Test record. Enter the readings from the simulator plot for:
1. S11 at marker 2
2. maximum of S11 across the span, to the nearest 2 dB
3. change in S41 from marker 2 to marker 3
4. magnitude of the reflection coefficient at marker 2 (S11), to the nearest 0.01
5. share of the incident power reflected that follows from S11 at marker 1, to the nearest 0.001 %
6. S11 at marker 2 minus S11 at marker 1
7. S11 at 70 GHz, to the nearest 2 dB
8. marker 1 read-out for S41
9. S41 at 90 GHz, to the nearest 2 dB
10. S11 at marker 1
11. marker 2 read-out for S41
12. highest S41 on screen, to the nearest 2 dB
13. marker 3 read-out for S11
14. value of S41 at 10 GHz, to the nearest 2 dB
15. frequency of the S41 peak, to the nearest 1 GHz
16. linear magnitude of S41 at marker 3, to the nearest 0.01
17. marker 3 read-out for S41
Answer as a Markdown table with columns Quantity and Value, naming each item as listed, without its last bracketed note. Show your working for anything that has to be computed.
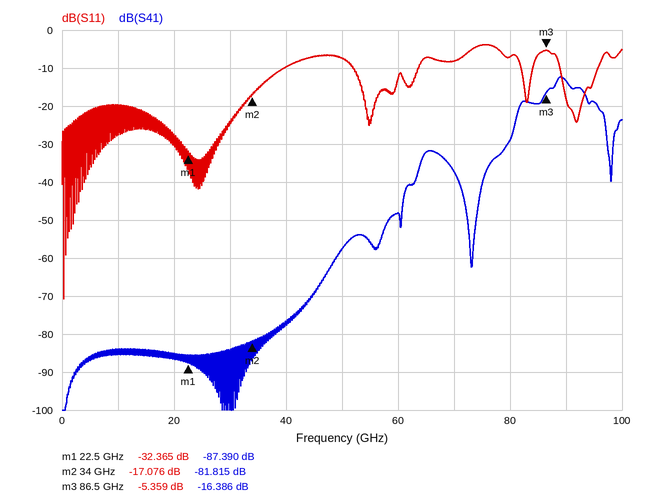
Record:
| Quantity | Value |
|---|---|
| S11 at marker 2 | -17.076 dB |
| maximum of S11 across the span, to the nearest 2 dB | -4 dB |
| change in S41 from marker 2 to marker 3 | -16.386 − (-81.815) = 65.429 dB |
| magnitude of the reflection coefficient at marker 2 (S11), to the nearest 0.01 | 10^(-17.076/20) ≈ 0.14 |
| share of the incident power reflected that follows from S11 at marker 1, to the nearest 0.001 % | 10^(-32.365/10) ≈ 0.058 % |
| S11 at marker 2 minus S11 at marker 1 | -17.076 − (-32.365) = 15.289 dB |
| S11 at 70 GHz, to the nearest 2 dB | -8 dB |
| marker 1 read-out for S41 | -87.390 dB |
| S41 at 90 GHz, to the nearest 2 dB | -14 dB |
| S11 at marker 1 | -32.365 dB |
| marker 2 read-out for S41 | -81.815 dB |
| highest S41 on screen, to the nearest 2 dB | -12 dB |
| marker 3 read-out for S11 | -5.359 dB |
| value of S41 at 10 GHz, to the nearest 2 dB | -84 dB |
| frequency of the S41 peak, to the nearest 1 GHz | 89 GHz |
| linear magnitude of S41 at marker 3, to the nearest 0.01 | 10^(-16.386/20) ≈ 0.15 |
| marker 3 read-out for S41 | -16.386 dB |
